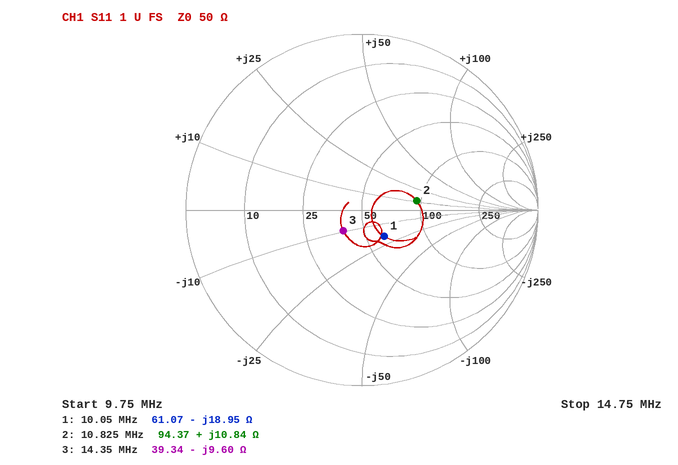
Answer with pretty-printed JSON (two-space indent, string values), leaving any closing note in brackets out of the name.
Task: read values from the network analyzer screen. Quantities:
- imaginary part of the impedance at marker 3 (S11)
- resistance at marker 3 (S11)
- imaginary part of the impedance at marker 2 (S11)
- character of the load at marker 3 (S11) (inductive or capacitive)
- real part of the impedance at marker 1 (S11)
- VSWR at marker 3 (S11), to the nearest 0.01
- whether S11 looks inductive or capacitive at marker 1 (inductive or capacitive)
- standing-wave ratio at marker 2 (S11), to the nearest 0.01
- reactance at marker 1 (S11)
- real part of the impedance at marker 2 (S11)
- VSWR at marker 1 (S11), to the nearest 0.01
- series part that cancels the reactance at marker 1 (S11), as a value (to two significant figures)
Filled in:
{
  "imaginary part of the impedance at marker 3": "-9.60 Ω",
  "resistance at marker 3": "39.34 Ω",
  "imaginary part of the impedance at marker 2": "+10.84 Ω",
  "character of the load at marker 3 (S11)": "capacitive",
  "real part of the impedance at marker 1": "61.07 Ω",
  "VSWR at marker 3 (S11), to the nearest 0.01": "1.38",
  "whether S11 looks inductive or capacitive at marker 1": "capacitive",
  "standing-wave ratio at marker 2 (S11), to the nearest 0.01": "1.92",
  "reactance at marker 1": "-18.95 Ω",
  "real part of the impedance at marker 2": "94.37 Ω",
  "VSWR at marker 1 (S11), to the nearest 0.01": "1.48",
  "series part that cancels the reactance at marker 1 (S11), as a value": "300 nH"
}
